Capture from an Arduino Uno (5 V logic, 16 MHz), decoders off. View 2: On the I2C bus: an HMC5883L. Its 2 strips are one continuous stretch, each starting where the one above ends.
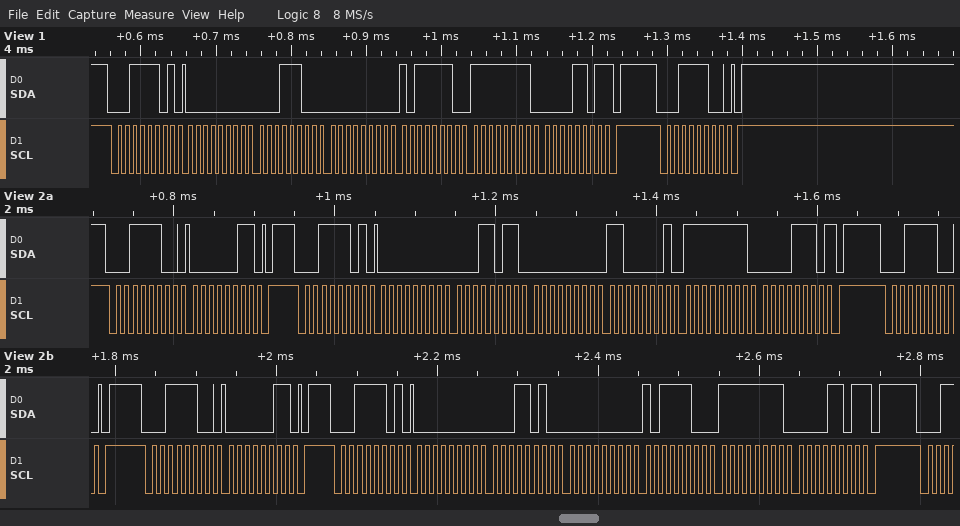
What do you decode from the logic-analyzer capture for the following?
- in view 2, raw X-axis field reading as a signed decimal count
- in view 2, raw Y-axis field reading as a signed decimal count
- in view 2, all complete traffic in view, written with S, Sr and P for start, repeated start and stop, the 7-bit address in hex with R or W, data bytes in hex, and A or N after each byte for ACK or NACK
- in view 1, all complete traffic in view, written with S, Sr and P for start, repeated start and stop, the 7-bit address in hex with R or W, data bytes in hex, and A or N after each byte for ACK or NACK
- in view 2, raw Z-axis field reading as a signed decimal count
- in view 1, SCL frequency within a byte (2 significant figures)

27
-242
S 1EW A 03 A P S 1ER A 00 A 1B A 00 A C1 A FF A 0E N P S 1EW A P S 1EW A 03 A P S 1ER A 00 A 1A A 00 A BC A FF A 0D N P
S 1ER A 00 A 1C A 00 A BE A FF A 0D N P S 1EW A P
193
100 kHz
